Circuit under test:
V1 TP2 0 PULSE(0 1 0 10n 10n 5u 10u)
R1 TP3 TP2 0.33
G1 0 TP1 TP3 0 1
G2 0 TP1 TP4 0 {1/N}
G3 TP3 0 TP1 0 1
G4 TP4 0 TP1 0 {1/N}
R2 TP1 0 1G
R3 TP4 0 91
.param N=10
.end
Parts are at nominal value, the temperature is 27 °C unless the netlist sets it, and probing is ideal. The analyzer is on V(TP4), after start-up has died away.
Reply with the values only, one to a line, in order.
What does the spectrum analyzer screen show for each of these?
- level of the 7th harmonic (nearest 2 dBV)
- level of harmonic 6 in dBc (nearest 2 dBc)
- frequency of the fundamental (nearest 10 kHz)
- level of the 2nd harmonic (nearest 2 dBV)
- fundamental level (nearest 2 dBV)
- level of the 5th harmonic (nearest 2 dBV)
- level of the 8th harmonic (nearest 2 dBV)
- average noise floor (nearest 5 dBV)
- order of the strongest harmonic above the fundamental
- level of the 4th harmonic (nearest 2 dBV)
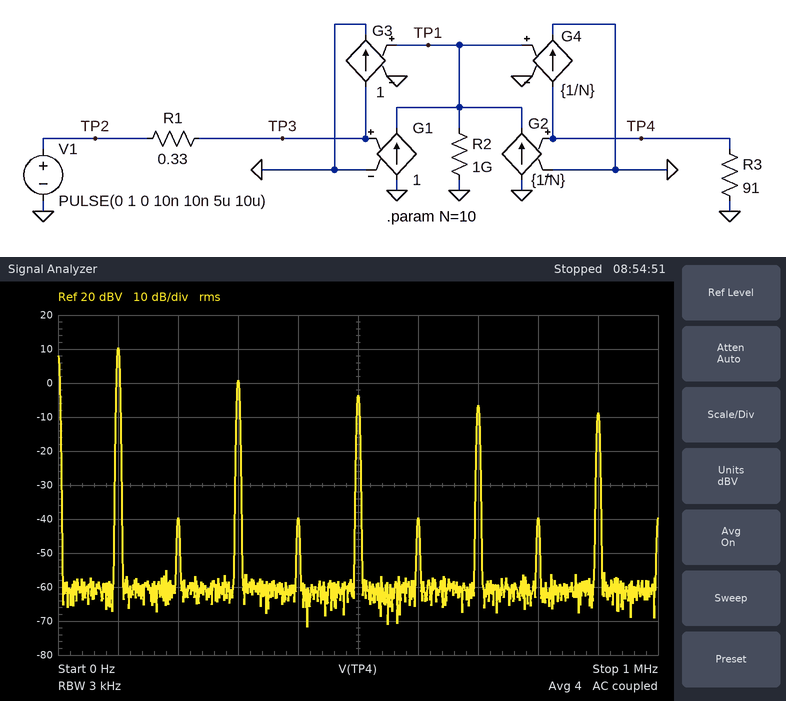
-6 dBV
-50 dBc
100 kHz
-40 dBV
10 dBV
-4 dBV
-40 dBV
-60 dBV
3
-40 dBV
